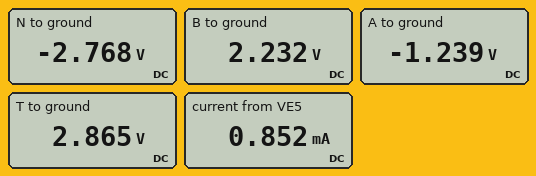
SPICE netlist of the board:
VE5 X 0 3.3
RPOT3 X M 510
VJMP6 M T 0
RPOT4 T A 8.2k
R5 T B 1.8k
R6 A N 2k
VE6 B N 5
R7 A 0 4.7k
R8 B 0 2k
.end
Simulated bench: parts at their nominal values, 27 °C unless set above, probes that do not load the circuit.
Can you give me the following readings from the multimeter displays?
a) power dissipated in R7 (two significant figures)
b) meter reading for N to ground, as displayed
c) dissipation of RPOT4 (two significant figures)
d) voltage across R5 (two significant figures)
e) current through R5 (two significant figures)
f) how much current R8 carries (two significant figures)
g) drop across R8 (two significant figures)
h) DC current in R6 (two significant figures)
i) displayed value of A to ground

330 µW
-2.768 V
2.1 mW
630 mV
350 µA
1.1 mA
2.2 V
760 µA
-1.239 V
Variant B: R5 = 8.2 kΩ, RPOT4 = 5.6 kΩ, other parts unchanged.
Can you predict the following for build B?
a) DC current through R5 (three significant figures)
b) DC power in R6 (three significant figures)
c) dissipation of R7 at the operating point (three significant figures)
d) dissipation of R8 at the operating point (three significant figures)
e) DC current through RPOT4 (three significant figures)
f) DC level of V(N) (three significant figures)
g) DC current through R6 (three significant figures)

100 µA
1.74 mW
242 µW
2.14 mW
706 µA
-2.93 V
933 µA
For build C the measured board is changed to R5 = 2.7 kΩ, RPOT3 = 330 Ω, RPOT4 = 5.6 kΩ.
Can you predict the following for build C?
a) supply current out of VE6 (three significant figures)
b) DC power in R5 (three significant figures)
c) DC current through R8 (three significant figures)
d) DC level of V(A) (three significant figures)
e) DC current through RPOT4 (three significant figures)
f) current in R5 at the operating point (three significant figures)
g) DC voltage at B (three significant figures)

893 µA
176 µW
1.15 mA
-919 mV
697 µA
255 µA
2.30 V
